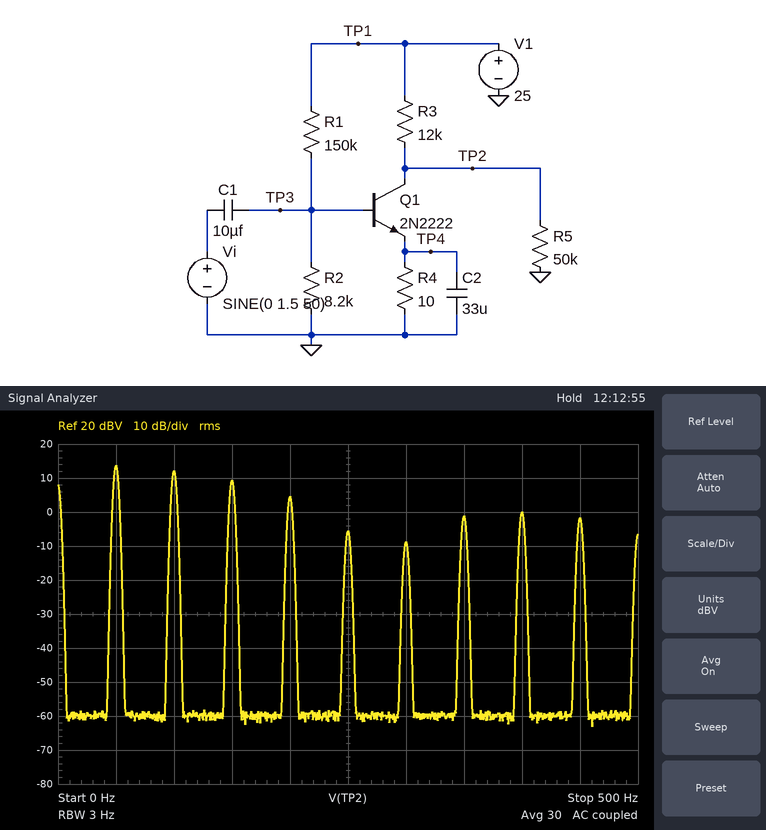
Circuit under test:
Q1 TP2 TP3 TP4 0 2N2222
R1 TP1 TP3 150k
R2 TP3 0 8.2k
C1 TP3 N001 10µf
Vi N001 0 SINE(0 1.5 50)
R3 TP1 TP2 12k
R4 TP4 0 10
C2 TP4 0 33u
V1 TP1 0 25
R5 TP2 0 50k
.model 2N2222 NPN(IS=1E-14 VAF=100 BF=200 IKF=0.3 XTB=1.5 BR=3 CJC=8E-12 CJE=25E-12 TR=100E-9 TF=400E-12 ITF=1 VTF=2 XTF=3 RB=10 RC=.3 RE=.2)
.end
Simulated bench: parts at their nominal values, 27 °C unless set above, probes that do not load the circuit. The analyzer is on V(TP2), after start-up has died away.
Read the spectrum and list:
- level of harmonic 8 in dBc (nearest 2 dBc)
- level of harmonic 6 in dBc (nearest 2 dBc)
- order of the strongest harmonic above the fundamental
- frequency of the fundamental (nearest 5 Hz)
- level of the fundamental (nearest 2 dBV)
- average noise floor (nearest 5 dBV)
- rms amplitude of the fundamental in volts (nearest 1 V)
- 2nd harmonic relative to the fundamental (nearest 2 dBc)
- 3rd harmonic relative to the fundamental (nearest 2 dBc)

-14 dBc
-22 dBc
2
50 Hz
14 dBV
-60 dBV
5 V
-2 dBc
-4 dBc
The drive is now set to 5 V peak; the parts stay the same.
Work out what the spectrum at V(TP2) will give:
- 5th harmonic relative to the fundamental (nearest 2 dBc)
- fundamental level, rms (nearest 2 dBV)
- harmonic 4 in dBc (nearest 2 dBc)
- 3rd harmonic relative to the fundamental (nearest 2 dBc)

-10 dBc
12 dBV
-6 dBc
-2 dBc
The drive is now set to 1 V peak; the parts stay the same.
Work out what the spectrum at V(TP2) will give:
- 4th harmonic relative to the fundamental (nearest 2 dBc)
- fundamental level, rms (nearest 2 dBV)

-12 dBc
14 dBV
